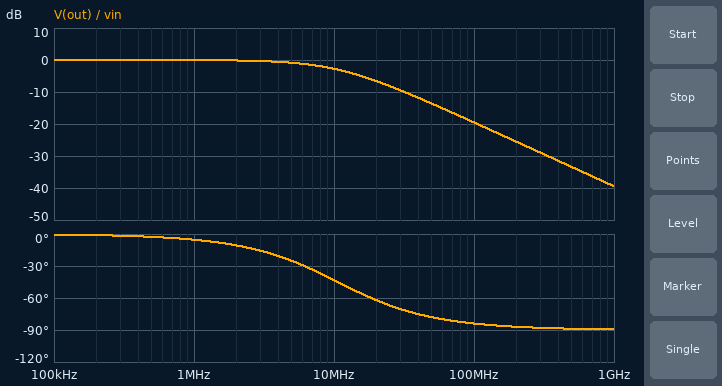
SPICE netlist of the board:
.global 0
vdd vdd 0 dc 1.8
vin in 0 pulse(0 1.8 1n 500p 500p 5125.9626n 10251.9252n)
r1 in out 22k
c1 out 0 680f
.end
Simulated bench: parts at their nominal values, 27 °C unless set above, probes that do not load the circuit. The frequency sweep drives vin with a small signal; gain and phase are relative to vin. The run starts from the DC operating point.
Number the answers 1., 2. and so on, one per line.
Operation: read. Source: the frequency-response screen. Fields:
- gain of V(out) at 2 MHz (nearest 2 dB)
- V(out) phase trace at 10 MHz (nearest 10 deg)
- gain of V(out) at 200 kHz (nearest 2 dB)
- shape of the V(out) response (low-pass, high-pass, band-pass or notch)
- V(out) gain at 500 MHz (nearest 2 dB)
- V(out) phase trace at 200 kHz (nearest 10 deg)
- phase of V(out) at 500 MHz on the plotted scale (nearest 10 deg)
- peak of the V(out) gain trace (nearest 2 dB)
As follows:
1. 0 dB
2. -40 deg
3. 0 dB
4. low-pass
5. -34 dB
6. 0 deg
7. -90 deg
8. 0 dB
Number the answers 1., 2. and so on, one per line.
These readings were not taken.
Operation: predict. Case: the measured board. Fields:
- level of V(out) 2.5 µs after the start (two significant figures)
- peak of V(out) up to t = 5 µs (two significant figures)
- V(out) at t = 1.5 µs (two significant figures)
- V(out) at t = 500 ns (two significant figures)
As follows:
1. 1.8 V
2. 1.8 V
3. 1.8 V
4. 1.8 V
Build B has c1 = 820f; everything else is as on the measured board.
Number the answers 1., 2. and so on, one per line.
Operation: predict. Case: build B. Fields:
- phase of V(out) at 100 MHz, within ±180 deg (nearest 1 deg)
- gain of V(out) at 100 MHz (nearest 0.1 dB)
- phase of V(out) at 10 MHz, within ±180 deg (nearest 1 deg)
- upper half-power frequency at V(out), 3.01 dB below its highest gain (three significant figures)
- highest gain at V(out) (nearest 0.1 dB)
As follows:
1. -85 deg
2. -21.1 dB
3. -49 deg
4. 8.82 MHz
5. 0 dB
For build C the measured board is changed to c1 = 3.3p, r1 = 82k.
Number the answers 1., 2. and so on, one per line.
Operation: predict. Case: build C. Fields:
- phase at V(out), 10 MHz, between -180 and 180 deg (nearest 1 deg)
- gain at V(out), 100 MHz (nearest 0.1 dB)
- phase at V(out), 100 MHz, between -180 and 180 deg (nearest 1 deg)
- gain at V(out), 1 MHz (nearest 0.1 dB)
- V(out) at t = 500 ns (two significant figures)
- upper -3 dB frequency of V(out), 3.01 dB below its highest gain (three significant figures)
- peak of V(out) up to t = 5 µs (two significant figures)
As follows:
1. -87 deg
2. -44.6 dB
3. -90 deg
4. -5.9 dB
5. 1.5 V
6. 588 kHz
7. 1.8 V
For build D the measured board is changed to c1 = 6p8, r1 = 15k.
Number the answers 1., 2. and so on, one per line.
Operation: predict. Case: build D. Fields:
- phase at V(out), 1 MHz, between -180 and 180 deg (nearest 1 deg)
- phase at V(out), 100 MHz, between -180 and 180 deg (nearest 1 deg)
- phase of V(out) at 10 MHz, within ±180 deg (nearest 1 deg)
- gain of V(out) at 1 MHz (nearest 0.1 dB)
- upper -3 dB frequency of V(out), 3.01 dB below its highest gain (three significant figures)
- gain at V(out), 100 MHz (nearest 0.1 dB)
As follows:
1. -33 deg
2. -89 deg
3. -81 deg
4. -1.5 dB
5. 1.56 MHz
6. -36.1 dB
